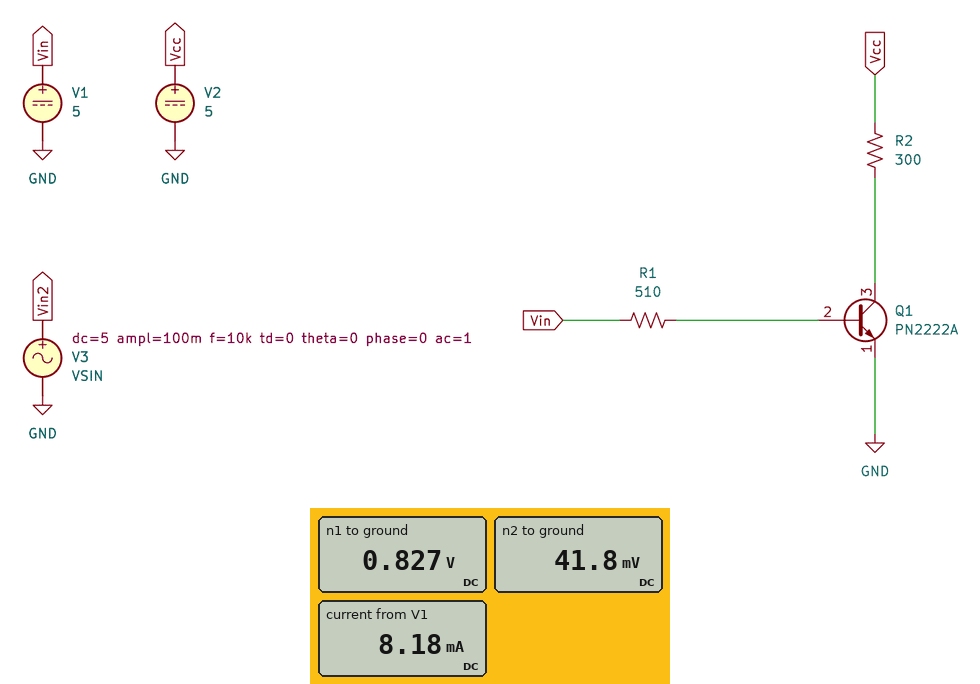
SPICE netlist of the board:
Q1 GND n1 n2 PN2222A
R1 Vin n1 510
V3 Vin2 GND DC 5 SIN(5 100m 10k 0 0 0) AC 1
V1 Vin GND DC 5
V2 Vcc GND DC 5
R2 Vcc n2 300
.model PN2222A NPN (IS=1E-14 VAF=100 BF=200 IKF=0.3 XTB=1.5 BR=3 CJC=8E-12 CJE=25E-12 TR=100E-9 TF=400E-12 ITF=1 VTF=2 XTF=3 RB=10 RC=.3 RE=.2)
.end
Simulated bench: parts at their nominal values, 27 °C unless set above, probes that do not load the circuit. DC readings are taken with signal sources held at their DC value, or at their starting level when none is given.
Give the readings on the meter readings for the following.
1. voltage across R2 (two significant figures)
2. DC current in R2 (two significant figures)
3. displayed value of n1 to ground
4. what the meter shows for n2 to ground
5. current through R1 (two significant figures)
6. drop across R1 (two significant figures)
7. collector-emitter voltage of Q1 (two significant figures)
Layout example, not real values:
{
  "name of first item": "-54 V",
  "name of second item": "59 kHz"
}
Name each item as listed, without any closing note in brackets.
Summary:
{
  "voltage across R2": "5.0 V",
  "DC current in R2": "17 mA",
  "displayed value of n1 to ground": "0.827 V",
  "what the meter shows for n2 to ground": "41.8 mV",
  "current through R1": "8.2 mA",
  "drop across R1": "4.2 V",
  "collector-emitter voltage of Q1": "-42 mV"
}
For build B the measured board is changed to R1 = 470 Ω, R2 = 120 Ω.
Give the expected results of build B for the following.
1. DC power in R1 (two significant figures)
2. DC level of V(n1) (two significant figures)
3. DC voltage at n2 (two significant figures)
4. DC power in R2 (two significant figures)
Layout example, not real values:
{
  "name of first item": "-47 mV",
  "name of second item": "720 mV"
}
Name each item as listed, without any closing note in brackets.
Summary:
{
  "DC power in R1": "37 mW",
  "DC level of V(n1)": "840 mV",
  "DC voltage at n2": "1.8 V",
  "DC power in R2": "83 mW"
}
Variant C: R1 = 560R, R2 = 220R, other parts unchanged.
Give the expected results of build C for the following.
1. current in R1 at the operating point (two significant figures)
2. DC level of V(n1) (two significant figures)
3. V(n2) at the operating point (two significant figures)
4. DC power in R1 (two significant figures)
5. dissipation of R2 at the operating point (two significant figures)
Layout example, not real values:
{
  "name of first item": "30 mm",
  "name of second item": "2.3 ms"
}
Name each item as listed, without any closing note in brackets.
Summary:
{
  "current in R1 at the operating point": "7.5 mA",
  "DC level of V(n1)": "820 mV",
  "V(n2) at the operating point": "140 mV",
  "DC power in R1": "31 mW",
  "dissipation of R2 at the operating point": "110 mW"
}
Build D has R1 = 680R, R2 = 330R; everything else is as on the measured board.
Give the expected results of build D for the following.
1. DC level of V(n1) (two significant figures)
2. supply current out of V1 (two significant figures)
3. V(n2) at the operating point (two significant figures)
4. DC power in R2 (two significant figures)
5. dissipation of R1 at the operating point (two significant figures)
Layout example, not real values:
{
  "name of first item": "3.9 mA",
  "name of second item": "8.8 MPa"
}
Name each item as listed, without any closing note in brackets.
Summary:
{
  "DC level of V(n1)": "800 mV",
  "supply current out of V1": "6.2 mA",
  "V(n2) at the operating point": "55 mV",
  "DC power in R2": "74 mW",
  "dissipation of R1 at the operating point": "26 mW"
}
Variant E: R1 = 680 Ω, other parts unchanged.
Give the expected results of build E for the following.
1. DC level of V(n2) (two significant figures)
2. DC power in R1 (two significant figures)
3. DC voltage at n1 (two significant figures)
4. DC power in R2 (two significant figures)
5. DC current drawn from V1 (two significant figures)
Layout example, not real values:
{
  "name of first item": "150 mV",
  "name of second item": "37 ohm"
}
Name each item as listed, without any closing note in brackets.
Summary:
{
  "DC level of V(n2)": "70 mV",
  "DC power in R1": "26 mW",
  "DC voltage at n1": "800 mV",
  "DC power in R2": "81 mW",
  "DC current drawn from V1": "6.2 mA"
}
